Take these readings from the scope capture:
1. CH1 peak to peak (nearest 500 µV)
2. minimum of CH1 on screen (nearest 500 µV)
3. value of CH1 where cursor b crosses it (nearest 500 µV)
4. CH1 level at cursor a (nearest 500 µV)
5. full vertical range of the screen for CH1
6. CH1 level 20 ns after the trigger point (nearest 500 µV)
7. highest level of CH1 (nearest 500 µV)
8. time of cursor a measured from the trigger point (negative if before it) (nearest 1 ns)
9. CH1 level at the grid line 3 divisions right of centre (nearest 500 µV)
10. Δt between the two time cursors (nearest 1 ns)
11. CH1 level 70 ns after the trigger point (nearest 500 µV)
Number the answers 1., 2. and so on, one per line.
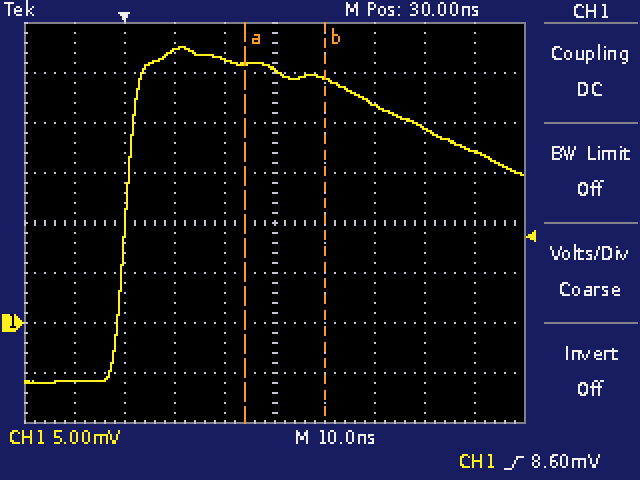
1. 33.5 mV
2. -6.0 mV
3. 24.5 mV
4. 26.0 mV
5. 40 mV
6. 26.5 mV
7. 27.5 mV
8. +24 ns
9. 19.5 mV
10. 16 ns
11. 17.0 mV
